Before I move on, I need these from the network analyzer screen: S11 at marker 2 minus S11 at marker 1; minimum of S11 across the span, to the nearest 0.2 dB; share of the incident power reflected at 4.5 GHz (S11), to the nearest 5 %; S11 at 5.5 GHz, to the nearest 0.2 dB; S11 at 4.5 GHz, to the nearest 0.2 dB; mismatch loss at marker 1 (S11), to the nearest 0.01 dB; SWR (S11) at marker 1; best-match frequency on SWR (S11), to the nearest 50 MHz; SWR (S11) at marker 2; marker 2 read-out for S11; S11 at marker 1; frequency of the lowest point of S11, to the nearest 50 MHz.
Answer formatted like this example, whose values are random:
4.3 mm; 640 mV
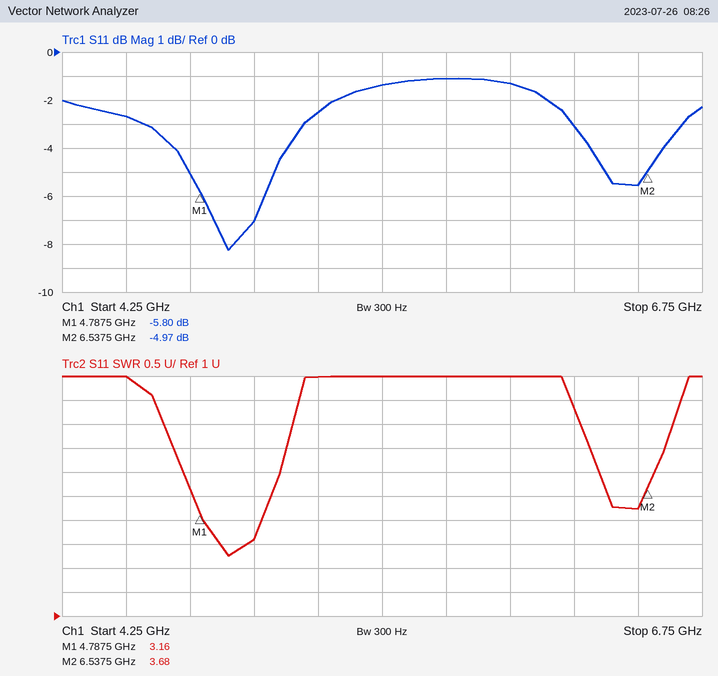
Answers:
0.83 dB; -8.2 dB; 55 %; -1.4 dB; -2.6 dB; 1.33 dB; 3.16; 4.90 GHz; 3.68; -4.97 dB; -5.80 dB; 4.90 GHz
